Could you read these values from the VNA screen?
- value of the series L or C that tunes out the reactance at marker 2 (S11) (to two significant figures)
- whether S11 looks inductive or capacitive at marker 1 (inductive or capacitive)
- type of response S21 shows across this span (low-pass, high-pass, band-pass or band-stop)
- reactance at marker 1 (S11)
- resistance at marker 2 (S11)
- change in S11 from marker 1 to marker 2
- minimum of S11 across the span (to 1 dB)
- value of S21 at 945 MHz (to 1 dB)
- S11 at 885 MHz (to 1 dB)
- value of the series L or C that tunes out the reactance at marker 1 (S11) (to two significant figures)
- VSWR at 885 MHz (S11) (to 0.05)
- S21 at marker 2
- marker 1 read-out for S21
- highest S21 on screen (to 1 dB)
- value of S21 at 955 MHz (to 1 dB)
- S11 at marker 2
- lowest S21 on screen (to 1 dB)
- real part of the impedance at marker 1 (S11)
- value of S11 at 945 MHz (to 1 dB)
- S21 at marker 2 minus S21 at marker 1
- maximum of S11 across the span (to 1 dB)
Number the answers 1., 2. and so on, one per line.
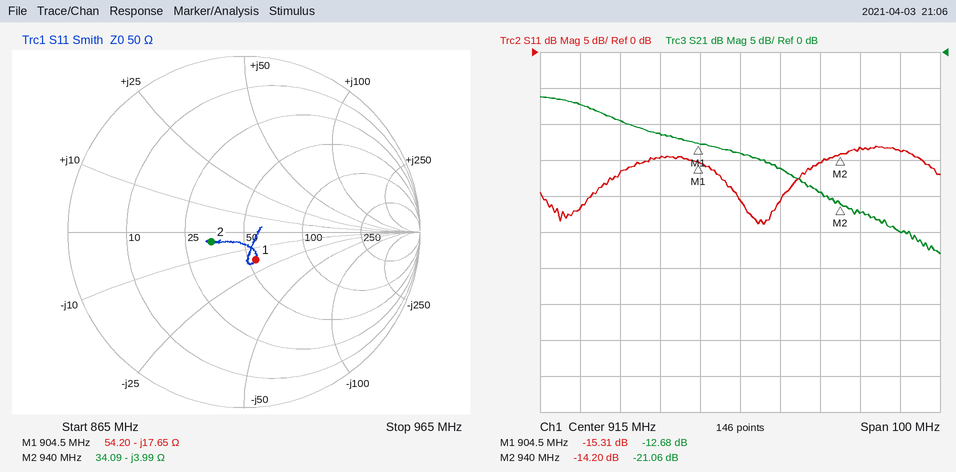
1. 680 pH
2. capacitive
3. low-pass
4. -17.65 Ω
5. 34.09 Ω
6. 1.11 dB
7. -24 dB
8. -22 dB
9. -17 dB
10. 3.1 nH
11. 1.35
12. -21.06 dB
13. -12.68 dB
14. -6 dB
15. -25 dB
16. -14.20 dB
17. -28 dB
18. 54.20 Ω
19. -13 dB
20. -8.38 dB
21. -13 dB
